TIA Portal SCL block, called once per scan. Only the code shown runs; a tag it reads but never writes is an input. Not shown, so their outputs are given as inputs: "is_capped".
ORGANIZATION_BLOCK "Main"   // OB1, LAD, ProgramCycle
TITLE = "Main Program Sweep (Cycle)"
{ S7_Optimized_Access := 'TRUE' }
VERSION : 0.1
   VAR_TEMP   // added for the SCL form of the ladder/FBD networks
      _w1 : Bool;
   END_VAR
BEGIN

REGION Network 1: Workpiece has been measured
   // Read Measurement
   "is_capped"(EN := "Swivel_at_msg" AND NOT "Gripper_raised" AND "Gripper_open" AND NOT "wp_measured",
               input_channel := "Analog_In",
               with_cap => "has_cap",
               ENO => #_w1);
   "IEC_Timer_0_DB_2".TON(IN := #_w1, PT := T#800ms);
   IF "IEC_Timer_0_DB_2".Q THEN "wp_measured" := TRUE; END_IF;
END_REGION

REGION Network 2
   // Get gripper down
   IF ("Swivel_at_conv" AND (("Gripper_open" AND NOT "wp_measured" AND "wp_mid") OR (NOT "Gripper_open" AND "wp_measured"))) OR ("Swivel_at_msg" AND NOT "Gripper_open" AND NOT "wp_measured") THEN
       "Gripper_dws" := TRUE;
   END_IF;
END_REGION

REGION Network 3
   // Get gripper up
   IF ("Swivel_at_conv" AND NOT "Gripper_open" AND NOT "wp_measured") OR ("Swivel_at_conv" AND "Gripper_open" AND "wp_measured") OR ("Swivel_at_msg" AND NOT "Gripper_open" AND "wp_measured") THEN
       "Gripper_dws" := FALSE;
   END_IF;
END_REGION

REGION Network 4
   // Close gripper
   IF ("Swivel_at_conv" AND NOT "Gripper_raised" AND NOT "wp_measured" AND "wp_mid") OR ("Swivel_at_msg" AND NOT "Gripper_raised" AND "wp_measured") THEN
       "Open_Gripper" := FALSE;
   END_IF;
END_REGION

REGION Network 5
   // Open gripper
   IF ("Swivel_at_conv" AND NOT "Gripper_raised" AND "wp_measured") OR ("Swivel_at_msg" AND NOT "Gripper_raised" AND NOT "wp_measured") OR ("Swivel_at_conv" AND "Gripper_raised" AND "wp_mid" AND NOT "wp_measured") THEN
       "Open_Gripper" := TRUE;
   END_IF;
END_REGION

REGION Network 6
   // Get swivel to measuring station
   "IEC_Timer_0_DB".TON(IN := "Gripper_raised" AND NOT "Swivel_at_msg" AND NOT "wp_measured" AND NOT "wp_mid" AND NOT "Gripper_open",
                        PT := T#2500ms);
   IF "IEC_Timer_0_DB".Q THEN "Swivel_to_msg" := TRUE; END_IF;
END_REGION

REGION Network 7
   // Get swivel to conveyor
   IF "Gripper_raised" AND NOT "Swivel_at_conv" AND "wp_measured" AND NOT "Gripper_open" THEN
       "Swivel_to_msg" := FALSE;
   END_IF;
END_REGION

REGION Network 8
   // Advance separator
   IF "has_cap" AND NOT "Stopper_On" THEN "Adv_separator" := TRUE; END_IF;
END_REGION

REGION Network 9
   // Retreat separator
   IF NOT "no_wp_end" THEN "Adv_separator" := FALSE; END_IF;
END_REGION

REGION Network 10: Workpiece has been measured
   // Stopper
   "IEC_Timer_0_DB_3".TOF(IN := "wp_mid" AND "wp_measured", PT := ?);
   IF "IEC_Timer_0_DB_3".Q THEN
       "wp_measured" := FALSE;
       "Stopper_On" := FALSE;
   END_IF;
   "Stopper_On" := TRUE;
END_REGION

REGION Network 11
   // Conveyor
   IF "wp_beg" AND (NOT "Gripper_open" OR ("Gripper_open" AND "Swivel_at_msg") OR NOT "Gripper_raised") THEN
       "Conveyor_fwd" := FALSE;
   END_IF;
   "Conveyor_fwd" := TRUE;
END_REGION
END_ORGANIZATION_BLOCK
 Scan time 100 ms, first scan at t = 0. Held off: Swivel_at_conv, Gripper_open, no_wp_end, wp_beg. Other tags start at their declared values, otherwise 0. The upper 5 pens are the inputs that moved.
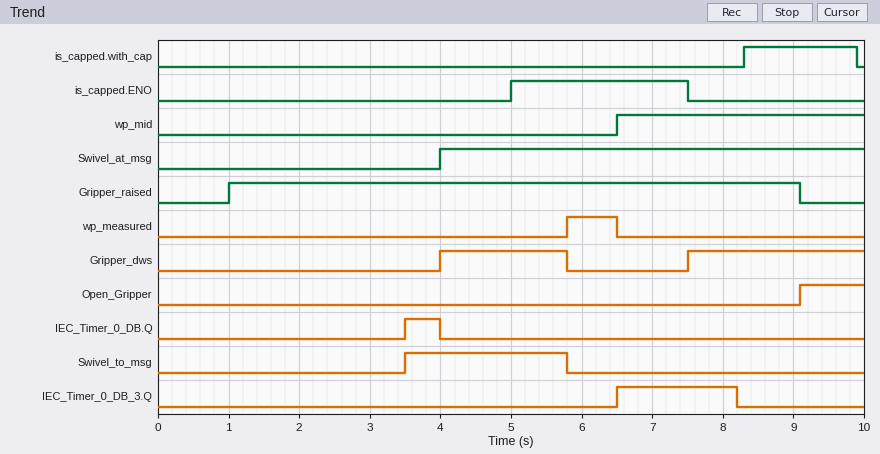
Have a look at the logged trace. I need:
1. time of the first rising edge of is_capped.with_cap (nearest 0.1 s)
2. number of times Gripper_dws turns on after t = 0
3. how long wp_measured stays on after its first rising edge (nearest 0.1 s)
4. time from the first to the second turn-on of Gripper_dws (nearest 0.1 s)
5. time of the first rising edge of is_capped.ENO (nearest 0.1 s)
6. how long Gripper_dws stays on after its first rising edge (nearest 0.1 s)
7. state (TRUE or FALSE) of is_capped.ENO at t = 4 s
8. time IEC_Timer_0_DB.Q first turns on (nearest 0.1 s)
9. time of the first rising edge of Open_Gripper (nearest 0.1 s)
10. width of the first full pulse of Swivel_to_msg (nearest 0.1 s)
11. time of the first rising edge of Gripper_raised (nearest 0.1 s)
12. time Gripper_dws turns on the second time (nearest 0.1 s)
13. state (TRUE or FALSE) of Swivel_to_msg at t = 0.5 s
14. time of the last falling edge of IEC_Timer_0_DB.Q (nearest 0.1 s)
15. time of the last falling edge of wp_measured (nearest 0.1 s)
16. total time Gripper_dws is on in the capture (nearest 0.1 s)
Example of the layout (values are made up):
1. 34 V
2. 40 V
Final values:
1. 8.3 s
2. 2
3. 0.7 s
4. 3.5 s
5. 5.0 s
6. 1.8 s
7. FALSE
8. 3.5 s
9. 9.1 s
10. 2.3 s
11. 1.0 s
12. 7.5 s
13. FALSE
14. 4.0 s
15. 6.5 s
16. 4.3 s
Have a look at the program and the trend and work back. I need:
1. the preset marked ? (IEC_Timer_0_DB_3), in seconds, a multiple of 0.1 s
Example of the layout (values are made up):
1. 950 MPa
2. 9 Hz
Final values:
1. 0.7 s
